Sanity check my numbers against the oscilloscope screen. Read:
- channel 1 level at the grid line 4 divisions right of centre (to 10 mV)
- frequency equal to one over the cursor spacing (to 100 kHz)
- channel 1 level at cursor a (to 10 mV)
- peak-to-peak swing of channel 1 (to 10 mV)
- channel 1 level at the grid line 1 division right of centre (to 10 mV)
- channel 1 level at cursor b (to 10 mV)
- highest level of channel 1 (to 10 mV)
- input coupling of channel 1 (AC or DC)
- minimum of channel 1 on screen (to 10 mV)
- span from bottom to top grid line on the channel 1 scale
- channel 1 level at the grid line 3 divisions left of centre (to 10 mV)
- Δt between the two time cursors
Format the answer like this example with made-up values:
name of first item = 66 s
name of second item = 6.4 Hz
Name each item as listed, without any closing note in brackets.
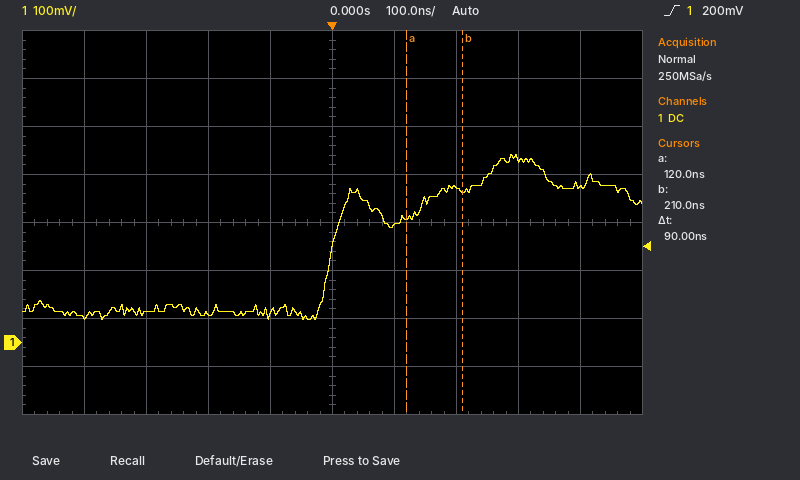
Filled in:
channel 1 level at the grid line 4 divisions right of centre = 320 mV
frequency equal to one over the cursor spacing = 11.1 MHz
channel 1 level at cursor a = 260 mV
peak-to-peak swing of channel 1 = 340 mV
channel 1 level at the grid line 1 division right of centre = 240 mV
channel 1 level at cursor b = 320 mV
highest level of channel 1 = 390 mV
input coupling of channel 1 = DC
minimum of channel 1 on screen = 50 mV
span from bottom to top grid line on the channel 1 scale = 800 mV
channel 1 level at the grid line 3 divisions left of centre = 60 mV
Δt between the two time cursors = 90 ns
